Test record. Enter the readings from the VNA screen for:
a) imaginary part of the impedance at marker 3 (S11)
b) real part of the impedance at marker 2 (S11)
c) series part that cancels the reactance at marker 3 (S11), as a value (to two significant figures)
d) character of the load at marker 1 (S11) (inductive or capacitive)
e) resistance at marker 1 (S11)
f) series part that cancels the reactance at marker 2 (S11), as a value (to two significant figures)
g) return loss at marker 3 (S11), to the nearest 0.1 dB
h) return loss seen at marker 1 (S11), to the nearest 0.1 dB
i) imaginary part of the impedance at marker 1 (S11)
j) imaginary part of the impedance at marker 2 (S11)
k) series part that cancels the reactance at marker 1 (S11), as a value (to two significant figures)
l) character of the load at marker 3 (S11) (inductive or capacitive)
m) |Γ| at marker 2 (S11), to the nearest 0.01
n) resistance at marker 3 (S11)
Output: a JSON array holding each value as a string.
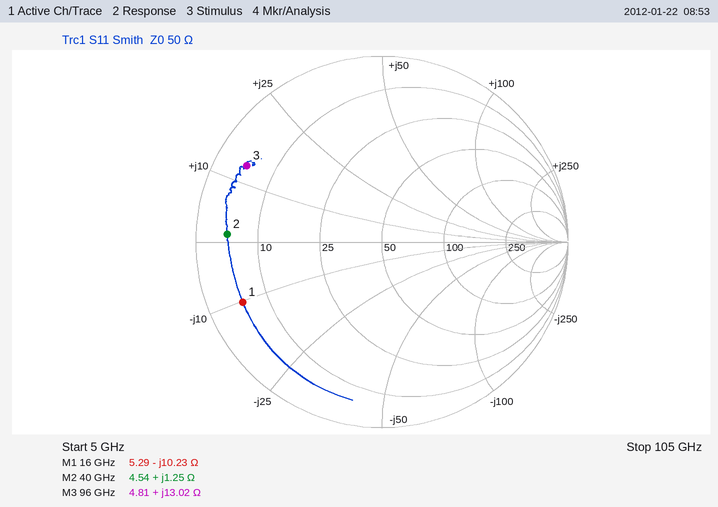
["+13.02 Ω", "4.54 Ω", "130 fF", "capacitive", "5.29 Ω", "3.2 pF", "1.6 dB", "1.8 dB", "-10.23 Ω", "+1.25 Ω", "100 pH", "inductive", "0.83", "4.81 Ω"]
